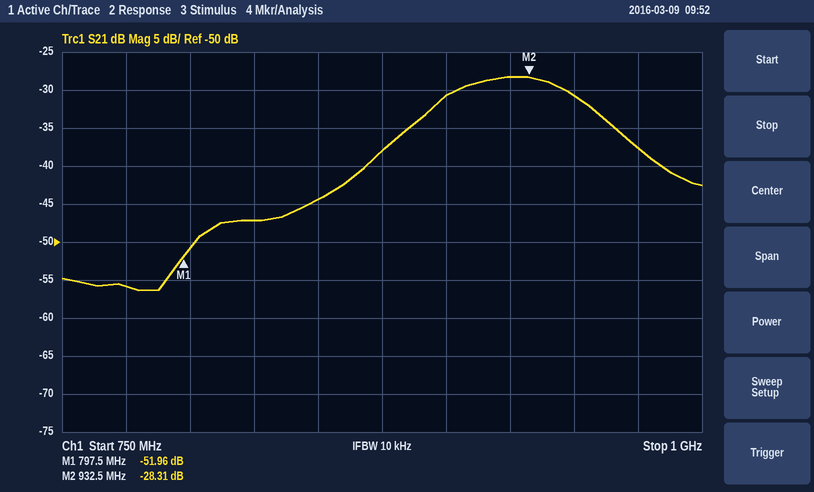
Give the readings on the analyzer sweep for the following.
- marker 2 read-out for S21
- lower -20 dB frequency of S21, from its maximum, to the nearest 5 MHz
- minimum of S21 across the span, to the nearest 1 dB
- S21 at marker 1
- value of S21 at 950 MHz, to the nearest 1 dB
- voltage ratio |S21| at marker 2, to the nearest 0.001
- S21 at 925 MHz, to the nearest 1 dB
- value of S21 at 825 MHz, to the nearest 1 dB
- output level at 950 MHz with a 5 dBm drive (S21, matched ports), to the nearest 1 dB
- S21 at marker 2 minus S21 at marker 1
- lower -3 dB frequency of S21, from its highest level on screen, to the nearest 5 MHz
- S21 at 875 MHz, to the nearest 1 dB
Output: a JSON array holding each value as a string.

["-28.31 dB", "810 MHz", "-56 dB", "-51.96 dB", "-31 dB", "0.038", "-28 dB", "-47 dB", "-26 dBm", "23.65 dB", "900 MHz", "-38 dB"]
